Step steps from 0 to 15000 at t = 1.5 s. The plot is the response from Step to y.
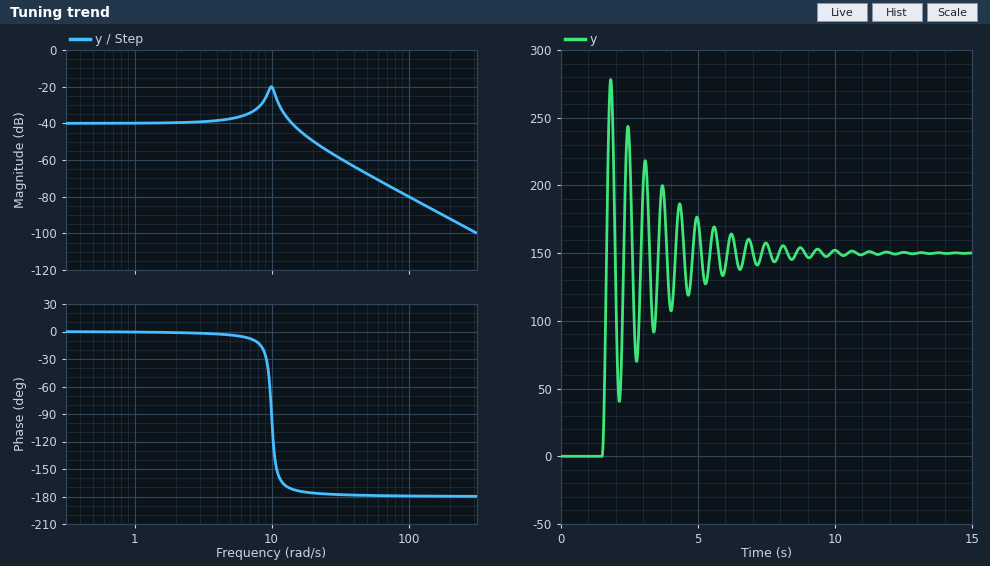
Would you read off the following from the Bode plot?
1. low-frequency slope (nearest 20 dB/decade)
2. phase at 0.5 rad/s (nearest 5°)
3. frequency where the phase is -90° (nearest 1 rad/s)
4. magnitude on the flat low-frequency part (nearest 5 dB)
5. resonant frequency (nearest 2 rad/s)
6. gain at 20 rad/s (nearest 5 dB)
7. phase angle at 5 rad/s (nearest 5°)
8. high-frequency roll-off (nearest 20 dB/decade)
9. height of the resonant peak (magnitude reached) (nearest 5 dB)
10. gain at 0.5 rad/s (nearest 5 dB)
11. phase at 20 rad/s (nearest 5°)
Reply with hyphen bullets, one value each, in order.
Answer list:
- 0 dB/decade
- 0°
- 10 rad/s
- -40 dB
- 10 rad/s
- -50 dB
- -5°
- -40 dB/decade
- -20 dB
- -40 dB
- -175°
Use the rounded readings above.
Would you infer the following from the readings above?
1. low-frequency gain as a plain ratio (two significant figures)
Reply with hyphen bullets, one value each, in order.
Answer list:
- 0.010
